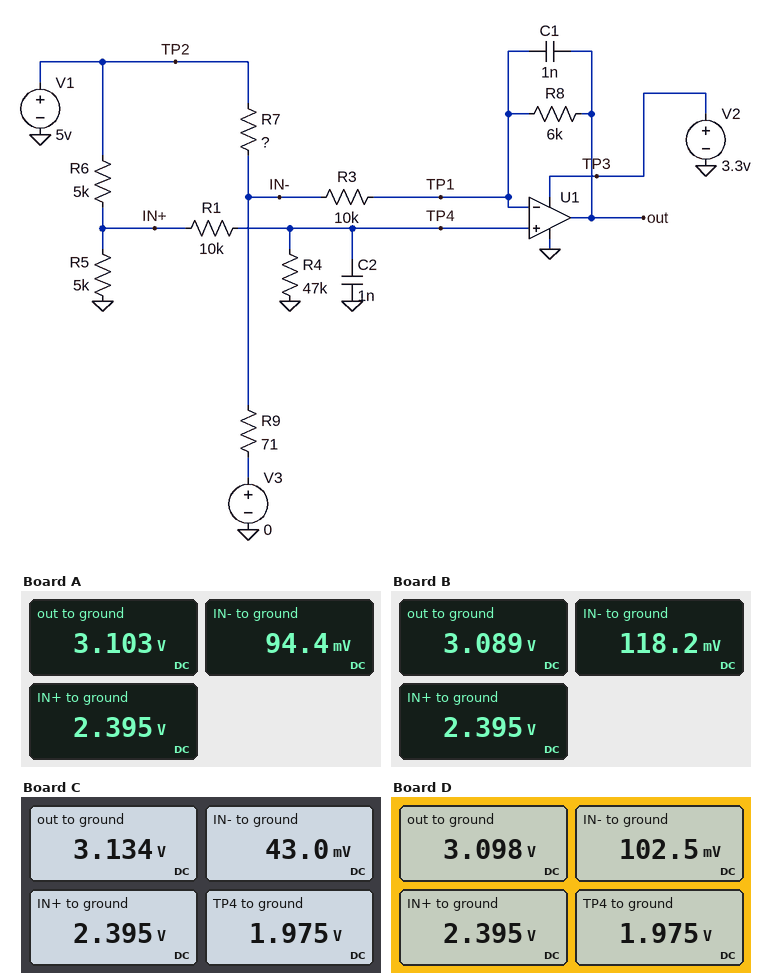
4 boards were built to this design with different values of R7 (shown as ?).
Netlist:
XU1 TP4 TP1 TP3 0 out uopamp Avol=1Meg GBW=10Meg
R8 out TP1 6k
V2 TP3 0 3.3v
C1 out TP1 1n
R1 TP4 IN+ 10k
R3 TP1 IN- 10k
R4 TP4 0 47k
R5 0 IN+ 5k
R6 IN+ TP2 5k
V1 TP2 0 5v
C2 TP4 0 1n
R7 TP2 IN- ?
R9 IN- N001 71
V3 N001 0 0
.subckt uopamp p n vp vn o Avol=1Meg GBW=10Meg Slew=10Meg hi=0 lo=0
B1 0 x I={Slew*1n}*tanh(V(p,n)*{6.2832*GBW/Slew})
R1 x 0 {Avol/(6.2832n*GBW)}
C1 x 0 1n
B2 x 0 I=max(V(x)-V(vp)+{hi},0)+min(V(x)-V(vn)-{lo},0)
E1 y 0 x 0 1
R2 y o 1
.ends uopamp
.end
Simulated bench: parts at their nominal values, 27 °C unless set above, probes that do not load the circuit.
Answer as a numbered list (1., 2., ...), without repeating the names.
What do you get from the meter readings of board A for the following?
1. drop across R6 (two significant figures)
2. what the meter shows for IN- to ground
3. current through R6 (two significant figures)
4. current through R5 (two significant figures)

1. 2.6 V
2. 94.4 mV
3. 520 µA
4. 480 µA
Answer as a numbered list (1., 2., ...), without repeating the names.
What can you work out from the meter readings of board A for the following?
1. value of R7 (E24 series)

1. 4.3 kΩ
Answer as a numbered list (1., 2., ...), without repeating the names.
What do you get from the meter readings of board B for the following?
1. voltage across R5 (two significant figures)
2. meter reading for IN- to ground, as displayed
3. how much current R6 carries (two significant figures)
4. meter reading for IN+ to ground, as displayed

1. 2.4 V
2. 118.2 mV
3. 520 µA
4. 2.395 V
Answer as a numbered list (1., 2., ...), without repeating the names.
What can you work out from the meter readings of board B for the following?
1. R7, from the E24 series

1. 3.3 kΩ
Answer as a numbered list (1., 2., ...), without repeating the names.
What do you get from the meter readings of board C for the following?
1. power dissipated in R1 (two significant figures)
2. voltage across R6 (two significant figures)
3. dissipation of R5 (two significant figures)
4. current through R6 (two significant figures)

1. 18 µW
2. 2.6 V
3. 1.1 mW
4. 520 µA
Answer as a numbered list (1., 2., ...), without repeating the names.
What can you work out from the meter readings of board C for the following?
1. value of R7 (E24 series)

1. 12 kΩ
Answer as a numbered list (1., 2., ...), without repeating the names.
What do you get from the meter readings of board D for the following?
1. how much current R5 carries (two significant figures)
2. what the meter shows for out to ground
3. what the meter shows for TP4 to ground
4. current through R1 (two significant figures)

1. 480 µA
2. 3.098 V
3. 1.975 V
4. 42 µA
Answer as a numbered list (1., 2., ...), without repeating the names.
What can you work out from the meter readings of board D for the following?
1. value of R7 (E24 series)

1. 3.9 kΩ
